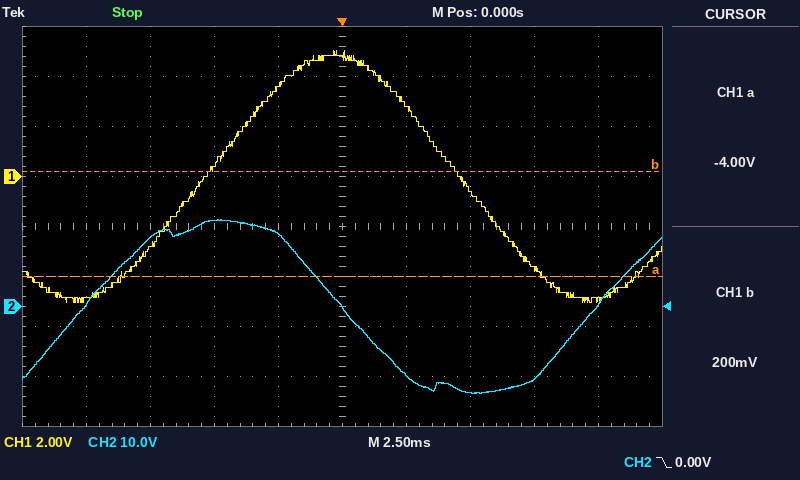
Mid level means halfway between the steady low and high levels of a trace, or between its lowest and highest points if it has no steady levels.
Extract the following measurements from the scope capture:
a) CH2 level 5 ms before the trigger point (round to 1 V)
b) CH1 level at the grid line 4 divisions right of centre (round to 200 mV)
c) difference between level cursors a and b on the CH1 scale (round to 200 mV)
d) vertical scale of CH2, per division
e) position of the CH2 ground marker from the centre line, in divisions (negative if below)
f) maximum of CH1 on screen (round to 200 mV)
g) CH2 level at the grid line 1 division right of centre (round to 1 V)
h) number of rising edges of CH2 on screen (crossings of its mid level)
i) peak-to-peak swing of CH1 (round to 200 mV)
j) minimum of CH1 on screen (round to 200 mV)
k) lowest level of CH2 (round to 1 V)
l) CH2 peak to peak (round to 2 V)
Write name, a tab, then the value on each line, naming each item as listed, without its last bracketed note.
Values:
CH2 level 5 ms before the trigger point	17 V
CH1 level at the grid line 4 divisions right of centre	-5.0 V
difference between level cursors a and b on the CH1 scale	4.2 V
vertical scale of CH2, per division	10 V
position of the CH2 ground marker from the centre line, in divisions	-1.6 div
maximum of CH1 on screen	5.0 V
CH2 level at the grid line 1 division right of centre	-14 V
number of rising edges of CH2 on screen	2
peak-to-peak swing of CH1	10.0 V
minimum of CH1 on screen	-5.0 V
lowest level of CH2	-17 V
CH2 peak to peak	34 V
